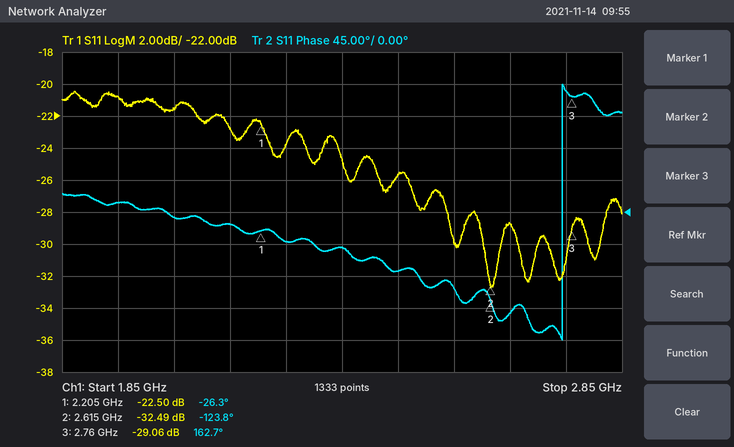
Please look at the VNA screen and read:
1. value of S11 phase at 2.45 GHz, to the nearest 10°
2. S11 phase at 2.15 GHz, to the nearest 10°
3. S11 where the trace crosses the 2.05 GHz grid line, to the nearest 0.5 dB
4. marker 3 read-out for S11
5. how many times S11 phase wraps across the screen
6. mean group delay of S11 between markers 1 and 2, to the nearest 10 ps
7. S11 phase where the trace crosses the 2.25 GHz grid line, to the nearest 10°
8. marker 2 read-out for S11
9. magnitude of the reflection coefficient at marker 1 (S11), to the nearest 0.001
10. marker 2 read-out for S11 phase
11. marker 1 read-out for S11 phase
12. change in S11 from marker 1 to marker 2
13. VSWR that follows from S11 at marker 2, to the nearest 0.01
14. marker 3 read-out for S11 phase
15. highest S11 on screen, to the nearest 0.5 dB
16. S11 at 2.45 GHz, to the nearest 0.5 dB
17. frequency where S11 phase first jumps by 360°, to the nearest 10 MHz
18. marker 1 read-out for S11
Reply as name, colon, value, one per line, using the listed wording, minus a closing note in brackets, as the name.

value of S11 phase at 2.45 GHz, to the nearest 10°: -80°
S11 phase at 2.15 GHz, to the nearest 10°: -20°
S11 where the trace crosses the 2.05 GHz grid line, to the nearest 0.5 dB: -21.5 dB
marker 3 read-out for S11: -29.06 dB
how many times S11 phase wraps across the screen: 1
mean group delay of S11 between markers 1 and 2, to the nearest 10 ps: 660 ps
S11 phase where the trace crosses the 2.25 GHz grid line, to the nearest 10°: -40°
marker 2 read-out for S11: -32.49 dB
magnitude of the reflection coefficient at marker 1 (S11), to the nearest 0.001: 0.075
marker 2 read-out for S11 phase: -123.8°
marker 1 read-out for S11 phase: -26.3°
change in S11 from marker 1 to marker 2: -9.99 dB
VSWR that follows from S11 at marker 2, to the nearest 0.01: 1.05
marker 3 read-out for S11 phase: 162.7°
highest S11 on screen, to the nearest 0.5 dB: -20.5 dB
S11 at 2.45 GHz, to the nearest 0.5 dB: -25.5 dB
frequency where S11 phase first jumps by 360°, to the nearest 10 MHz: 2.74 GHz
marker 1 read-out for S11: -22.50 dB
